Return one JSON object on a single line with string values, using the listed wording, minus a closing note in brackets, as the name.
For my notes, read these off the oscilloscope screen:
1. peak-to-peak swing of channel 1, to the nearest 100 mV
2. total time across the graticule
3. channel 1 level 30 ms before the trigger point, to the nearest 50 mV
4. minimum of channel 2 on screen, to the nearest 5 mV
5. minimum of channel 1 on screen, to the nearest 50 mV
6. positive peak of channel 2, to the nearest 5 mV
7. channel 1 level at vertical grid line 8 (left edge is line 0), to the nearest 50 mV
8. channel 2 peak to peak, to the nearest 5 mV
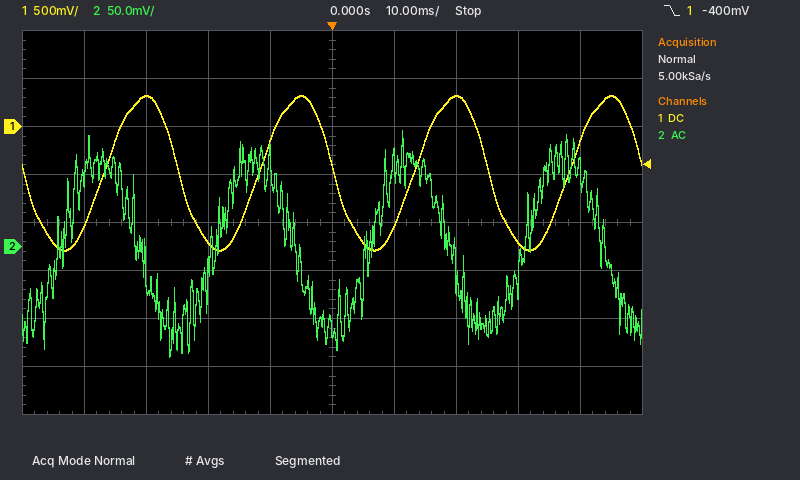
{"peak-to-peak swing of channel 1, to the nearest 100 mV": "1.60 V", "total time across the graticule": "100 ms", "channel 1 level 30 ms before the trigger point, to the nearest 50 mV": "300 mV", "minimum of channel 2 on screen, to the nearest 5 mV": "-115 mV", "minimum of channel 1 on screen, to the nearest 50 mV": "-1.30 V", "positive peak of channel 2, to the nearest 5 mV": "120 mV", "channel 1 level at vertical grid line 8 (left edge is line 0), to the nearest 50 mV": "-1.20 V", "channel 2 peak to peak, to the nearest 5 mV": "235 mV"}
